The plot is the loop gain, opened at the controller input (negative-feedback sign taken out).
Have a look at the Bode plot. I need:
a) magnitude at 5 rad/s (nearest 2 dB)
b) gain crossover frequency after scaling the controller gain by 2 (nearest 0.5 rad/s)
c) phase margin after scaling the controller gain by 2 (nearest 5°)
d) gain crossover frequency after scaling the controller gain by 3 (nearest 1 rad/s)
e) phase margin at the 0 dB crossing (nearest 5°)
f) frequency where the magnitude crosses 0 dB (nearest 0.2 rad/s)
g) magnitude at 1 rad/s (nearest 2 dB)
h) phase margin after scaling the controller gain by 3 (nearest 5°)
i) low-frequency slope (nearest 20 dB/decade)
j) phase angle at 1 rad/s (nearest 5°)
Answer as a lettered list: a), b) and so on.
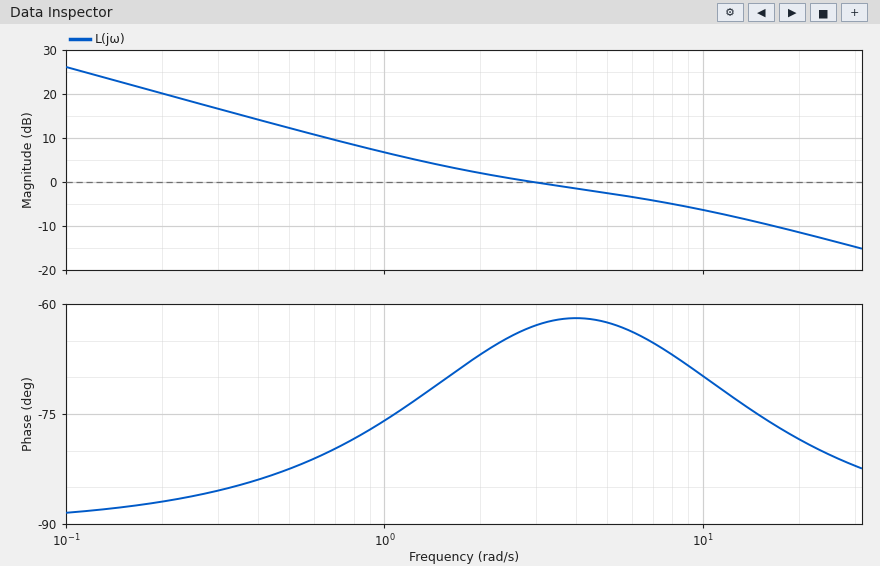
a) -2 dB
b) 9.5 rad/s
c) 110°
d) 16 rad/s
e) 115°
f) 3.0 rad/s
g) 6 dB
h) 105°
i) -20 dB/decade
j) -75°
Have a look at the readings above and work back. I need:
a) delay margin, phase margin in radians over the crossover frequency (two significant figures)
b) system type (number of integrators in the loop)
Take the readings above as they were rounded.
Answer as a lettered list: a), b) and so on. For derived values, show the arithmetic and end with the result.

a) 115 × π / 180 / 3 = 0.67 s
b) 1
